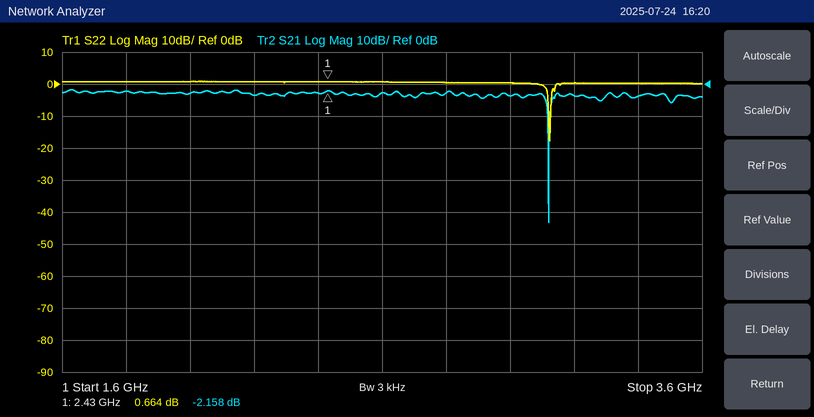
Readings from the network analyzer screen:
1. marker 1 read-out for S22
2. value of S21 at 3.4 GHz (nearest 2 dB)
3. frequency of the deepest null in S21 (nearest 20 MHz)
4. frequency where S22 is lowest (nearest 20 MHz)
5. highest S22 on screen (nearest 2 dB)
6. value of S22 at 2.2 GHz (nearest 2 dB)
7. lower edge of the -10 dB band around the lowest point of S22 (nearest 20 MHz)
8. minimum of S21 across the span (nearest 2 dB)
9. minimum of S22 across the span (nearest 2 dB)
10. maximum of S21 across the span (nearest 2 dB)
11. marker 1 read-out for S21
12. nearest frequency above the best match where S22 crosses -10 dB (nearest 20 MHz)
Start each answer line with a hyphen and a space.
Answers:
- 0.664 dB
- -4 dB
- 3.12 GHz
- 3.12 GHz
- 0 dB
- 0 dB
- 3.12 GHz
- -44 dB
- -18 dB
- -2 dB
- -2.158 dB
- 3.12 GHz
